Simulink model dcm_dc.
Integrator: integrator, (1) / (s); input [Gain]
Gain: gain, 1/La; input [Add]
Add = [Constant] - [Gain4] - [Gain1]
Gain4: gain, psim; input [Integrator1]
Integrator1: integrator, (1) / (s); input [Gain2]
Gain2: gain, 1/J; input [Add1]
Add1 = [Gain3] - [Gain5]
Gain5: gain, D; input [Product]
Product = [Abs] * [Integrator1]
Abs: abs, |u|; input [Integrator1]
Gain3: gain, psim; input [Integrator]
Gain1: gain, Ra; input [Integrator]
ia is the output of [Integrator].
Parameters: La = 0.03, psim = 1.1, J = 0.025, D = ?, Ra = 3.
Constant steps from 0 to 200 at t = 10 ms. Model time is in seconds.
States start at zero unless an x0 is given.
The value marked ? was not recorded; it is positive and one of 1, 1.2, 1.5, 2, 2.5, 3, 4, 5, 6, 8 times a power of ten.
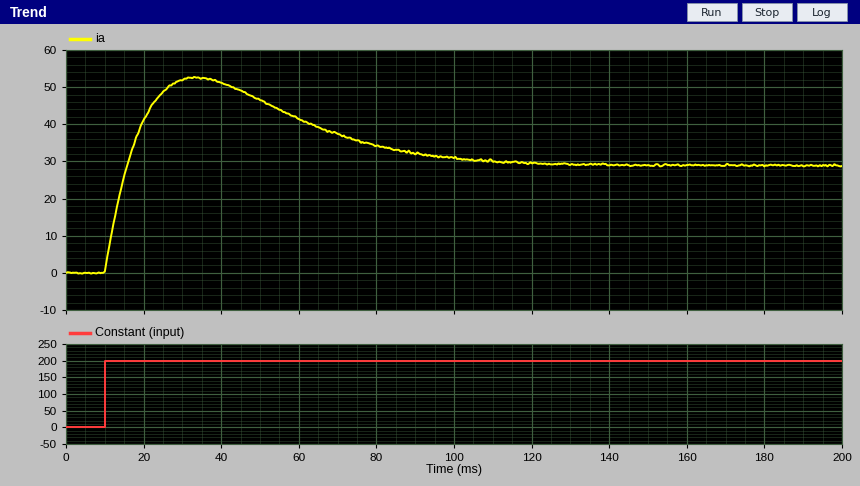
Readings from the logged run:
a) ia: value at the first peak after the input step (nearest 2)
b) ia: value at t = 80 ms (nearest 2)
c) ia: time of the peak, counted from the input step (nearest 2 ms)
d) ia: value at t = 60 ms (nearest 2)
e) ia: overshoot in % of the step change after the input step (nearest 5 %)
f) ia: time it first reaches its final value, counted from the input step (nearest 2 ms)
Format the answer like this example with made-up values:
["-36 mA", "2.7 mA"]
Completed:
["52", "34", "24 ms", "42", "80 %", "6 ms"]
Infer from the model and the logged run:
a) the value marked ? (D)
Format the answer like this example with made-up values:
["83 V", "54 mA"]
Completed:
["0.003"]
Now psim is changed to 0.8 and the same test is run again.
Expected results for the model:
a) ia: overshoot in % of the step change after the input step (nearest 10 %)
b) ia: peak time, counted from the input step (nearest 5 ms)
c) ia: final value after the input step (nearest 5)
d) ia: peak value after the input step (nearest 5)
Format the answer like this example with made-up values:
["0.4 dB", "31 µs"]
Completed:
["40 %", "30 ms", "40", "55"]
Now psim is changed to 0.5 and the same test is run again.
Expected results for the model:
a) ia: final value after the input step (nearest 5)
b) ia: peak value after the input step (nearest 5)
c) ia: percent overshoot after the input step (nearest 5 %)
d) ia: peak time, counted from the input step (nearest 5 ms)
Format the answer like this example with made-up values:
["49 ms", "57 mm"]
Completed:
["50", "60", "20 %", "35 ms"]
